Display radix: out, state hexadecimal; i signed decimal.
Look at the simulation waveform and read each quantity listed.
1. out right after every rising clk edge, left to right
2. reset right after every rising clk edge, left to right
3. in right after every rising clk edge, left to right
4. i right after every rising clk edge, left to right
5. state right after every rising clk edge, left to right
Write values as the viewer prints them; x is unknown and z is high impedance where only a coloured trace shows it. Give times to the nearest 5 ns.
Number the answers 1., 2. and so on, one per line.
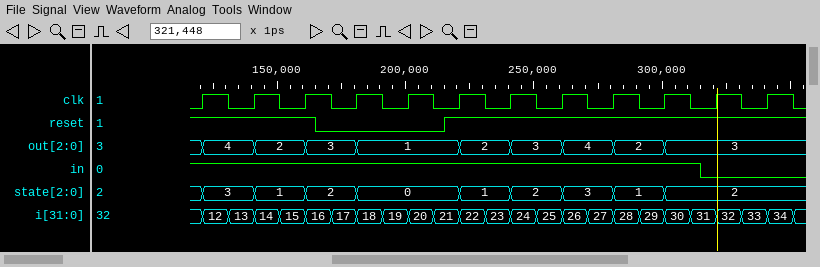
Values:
1. 4, 2, 3, 1, 1, 2, 3, 4, 2, 3, 3, 3
2. 1 1 1 0 0 1 1 1 1 1 1 1
3. 1 1 1 1 1 1 1 1 1 1 0 0
4. 12, 14, 16, 18, 20, 22, 24, 26, 28, 30, 32, 34
5. 3, 1, 2, 0, 0, 1, 2, 3, 1, 2, 2, 2
